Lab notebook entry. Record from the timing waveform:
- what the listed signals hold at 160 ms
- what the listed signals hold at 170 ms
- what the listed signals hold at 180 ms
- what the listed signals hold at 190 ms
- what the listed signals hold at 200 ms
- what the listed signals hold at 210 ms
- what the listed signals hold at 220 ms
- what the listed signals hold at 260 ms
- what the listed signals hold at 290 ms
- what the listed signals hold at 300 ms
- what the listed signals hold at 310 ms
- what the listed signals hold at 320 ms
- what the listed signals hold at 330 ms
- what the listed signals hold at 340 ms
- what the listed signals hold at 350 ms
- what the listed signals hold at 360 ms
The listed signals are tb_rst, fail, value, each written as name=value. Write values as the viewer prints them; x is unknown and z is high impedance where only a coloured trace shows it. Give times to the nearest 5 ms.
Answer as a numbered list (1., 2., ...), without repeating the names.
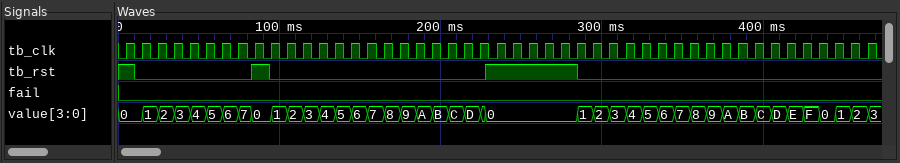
1. tb_rst=0, fail=0, value=7
2. tb_rst=0, fail=0, value=8
3. tb_rst=0, fail=0, value=9
4. tb_rst=0, fail=0, value=A
5. tb_rst=0, fail=0, value=B
6. tb_rst=0, fail=0, value=C
7. tb_rst=0, fail=0, value=D
8. tb_rst=1, fail=0, value=0
9. tb_rst=0, fail=0, value=1
10. tb_rst=0, fail=0, value=2
11. tb_rst=0, fail=0, value=3
12. tb_rst=0, fail=0, value=4
13. tb_rst=0, fail=0, value=5
14. tb_rst=0, fail=0, value=6
15. tb_rst=0, fail=0, value=7
16. tb_rst=0, fail=0, value=8
